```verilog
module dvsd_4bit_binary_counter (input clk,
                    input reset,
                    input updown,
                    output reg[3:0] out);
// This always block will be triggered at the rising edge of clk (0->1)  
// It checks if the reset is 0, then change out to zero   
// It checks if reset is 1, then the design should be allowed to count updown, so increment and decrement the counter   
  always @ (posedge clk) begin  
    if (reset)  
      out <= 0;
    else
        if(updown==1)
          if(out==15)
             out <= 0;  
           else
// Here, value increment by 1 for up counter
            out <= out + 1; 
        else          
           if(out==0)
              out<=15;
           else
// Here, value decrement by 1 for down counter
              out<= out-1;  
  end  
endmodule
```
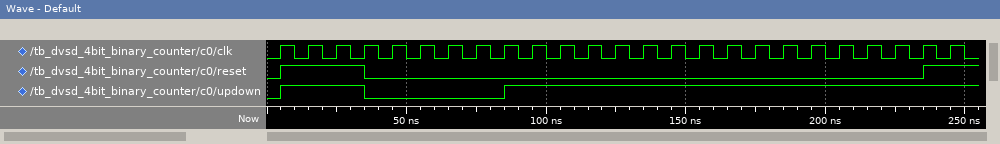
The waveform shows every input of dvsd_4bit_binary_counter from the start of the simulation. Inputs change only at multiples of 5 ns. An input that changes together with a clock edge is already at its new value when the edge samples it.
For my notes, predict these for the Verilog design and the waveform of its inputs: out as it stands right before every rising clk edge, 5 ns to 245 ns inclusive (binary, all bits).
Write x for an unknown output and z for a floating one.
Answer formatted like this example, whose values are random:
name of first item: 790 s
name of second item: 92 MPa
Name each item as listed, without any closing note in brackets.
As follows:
out as it stands right before every rising clk edge, 5 ns to 245 ns inclusive: x, 0000, 0000, 0000, 1111, 1110, 1101, 1100, 1011, 1100, 1101, 1110, 1111, 0000, 0001, 0010, 0011, 0100, 0101, 0110, 0111, 1000, 1001, 1010, 0000
